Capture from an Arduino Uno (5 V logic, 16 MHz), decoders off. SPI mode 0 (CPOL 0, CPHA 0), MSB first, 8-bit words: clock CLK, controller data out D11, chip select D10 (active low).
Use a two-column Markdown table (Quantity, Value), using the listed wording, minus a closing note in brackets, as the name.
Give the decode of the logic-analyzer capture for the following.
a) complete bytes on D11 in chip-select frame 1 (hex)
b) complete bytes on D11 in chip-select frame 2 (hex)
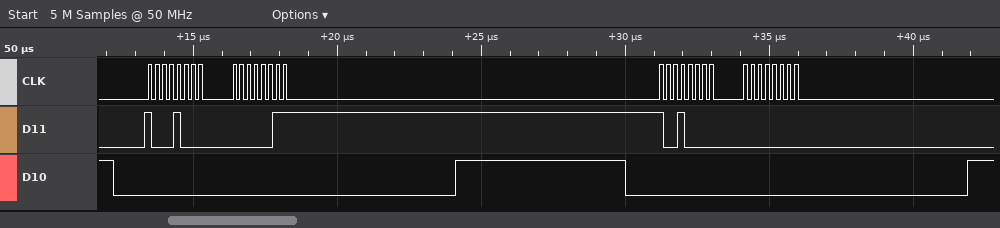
| Quantity | Value |
|---|---|
| complete bytes on D11 in chip-select frame 1 | 88 03 |
| complete bytes on D11 in chip-select frame 2 | 90 00 |
